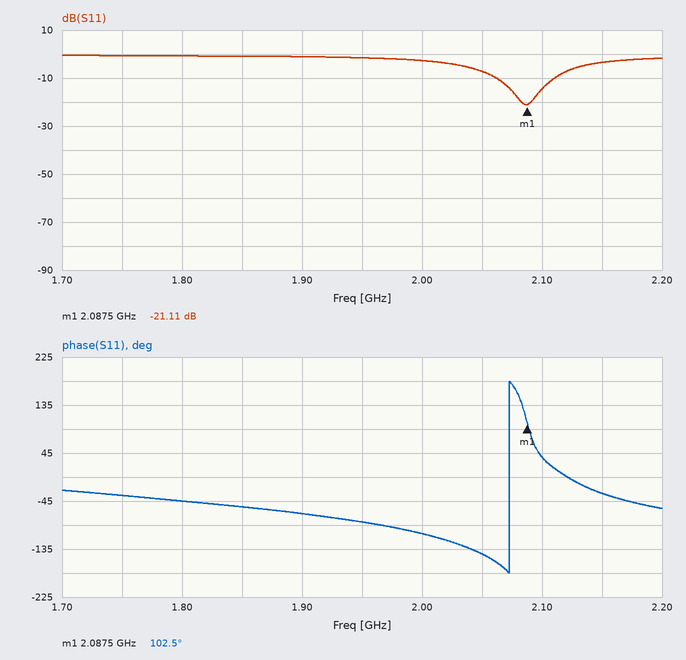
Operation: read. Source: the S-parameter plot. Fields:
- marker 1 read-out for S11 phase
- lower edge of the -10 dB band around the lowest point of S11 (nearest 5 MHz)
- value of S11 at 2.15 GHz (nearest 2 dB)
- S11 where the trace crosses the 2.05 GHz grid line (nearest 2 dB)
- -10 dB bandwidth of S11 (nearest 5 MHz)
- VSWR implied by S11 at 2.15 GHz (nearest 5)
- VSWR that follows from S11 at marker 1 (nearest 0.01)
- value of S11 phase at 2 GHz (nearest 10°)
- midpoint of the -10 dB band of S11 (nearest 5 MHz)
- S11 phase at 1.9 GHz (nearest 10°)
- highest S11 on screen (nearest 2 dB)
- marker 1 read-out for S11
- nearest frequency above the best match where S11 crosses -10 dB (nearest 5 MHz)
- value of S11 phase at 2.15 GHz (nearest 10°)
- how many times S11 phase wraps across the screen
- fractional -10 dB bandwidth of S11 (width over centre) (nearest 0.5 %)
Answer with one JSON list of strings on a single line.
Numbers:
["102.5°", "2.060 GHz", "-4 dB", "-8 dB", "50 MHz", "5", "1.19", "-110°", "2.085 GHz", "-70°", "0 dB", "-21.11 dB", "2.110 GHz", "-30°", "1", "2.5 %"]
